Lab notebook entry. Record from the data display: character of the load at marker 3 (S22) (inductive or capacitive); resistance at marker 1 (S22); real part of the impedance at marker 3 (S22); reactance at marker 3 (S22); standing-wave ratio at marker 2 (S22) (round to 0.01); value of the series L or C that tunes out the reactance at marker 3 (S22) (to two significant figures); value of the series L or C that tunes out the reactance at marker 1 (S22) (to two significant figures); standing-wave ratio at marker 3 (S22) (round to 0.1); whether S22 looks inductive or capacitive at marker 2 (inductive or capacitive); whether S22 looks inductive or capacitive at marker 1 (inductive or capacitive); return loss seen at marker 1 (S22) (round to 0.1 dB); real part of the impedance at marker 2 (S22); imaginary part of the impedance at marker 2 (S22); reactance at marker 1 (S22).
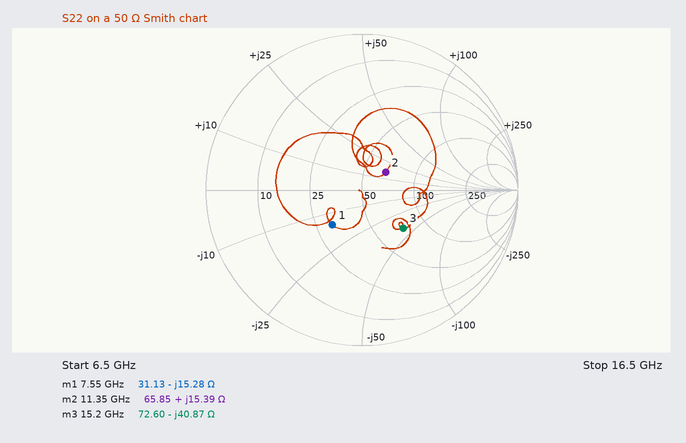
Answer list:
capacitive
31.13 Ω
72.60 Ω
-40.87 Ω
1.47
430 pH
320 pH
2.1
inductive
capacitive
10.6 dB
65.85 Ω
+15.39 Ω
-15.28 Ω
